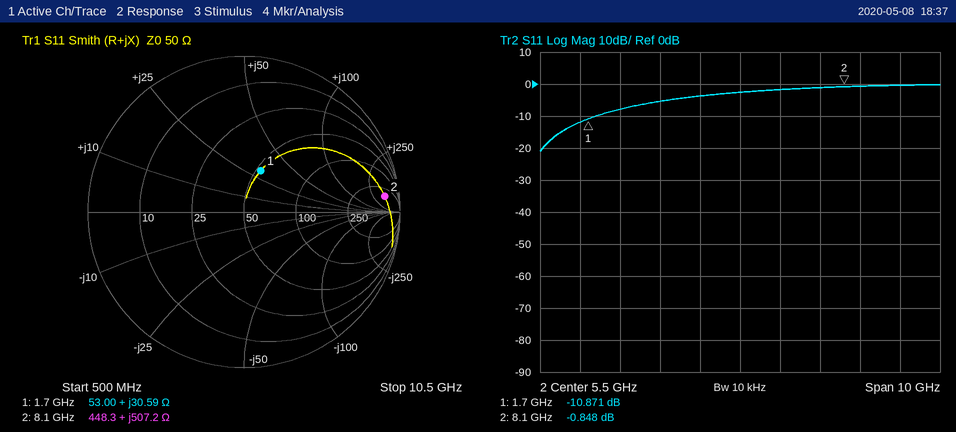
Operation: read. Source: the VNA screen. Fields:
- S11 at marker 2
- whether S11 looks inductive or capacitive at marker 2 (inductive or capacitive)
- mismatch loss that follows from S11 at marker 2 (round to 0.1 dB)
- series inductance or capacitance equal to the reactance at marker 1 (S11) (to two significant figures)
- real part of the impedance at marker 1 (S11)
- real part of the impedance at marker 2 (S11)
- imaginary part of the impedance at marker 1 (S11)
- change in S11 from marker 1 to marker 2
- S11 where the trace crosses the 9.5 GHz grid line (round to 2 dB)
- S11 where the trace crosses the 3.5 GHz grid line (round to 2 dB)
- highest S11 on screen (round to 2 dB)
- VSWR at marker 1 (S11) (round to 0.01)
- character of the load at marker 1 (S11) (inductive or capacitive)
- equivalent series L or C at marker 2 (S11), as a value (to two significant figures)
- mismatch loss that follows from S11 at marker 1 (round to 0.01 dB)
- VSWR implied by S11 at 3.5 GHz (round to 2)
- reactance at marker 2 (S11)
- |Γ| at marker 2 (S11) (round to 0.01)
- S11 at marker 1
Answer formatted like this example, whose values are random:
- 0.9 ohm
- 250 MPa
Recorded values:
- -0.848 dB
- inductive
- 7.5 dB
- 2.9 nH
- 53.00 Ω
- 448.3 Ω
- +30.59 Ω
- 10.023 dB
- 0 dB
- -6 dB
- 0 dB
- 1.80
- inductive
- 10.0 nH
- 0.37 dB
- 4
- +507.2 Ω
- 0.91
- -10.871 dB
